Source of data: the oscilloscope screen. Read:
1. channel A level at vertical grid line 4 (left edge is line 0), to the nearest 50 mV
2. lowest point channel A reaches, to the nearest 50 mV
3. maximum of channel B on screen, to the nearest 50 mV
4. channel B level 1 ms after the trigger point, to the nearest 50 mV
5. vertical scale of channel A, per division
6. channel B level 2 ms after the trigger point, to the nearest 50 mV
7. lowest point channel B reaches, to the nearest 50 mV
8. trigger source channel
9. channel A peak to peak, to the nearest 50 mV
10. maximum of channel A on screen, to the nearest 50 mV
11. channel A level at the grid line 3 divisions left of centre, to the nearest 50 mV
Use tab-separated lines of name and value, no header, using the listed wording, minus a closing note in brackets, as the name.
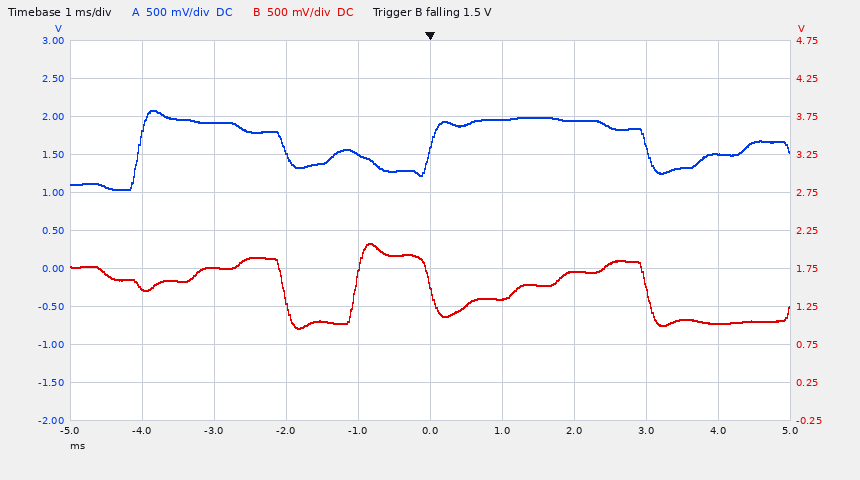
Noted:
channel A level at vertical grid line 4 (left edge is line 0), to the nearest 50 mV	1.50 V
lowest point channel A reaches, to the nearest 50 mV	1.05 V
maximum of channel B on screen, to the nearest 50 mV	2.10 V
channel B level 1 ms after the trigger point, to the nearest 50 mV	1.35 V
vertical scale of channel A, per division	500 mV
channel B level 2 ms after the trigger point, to the nearest 50 mV	1.70 V
lowest point channel B reaches, to the nearest 50 mV	950 mV
trigger source channel	channel B
channel A peak to peak, to the nearest 50 mV	1.05 V
maximum of channel A on screen, to the nearest 50 mV	2.10 V
channel A level at the grid line 3 divisions left of centre, to the nearest 50 mV	1.90 V
